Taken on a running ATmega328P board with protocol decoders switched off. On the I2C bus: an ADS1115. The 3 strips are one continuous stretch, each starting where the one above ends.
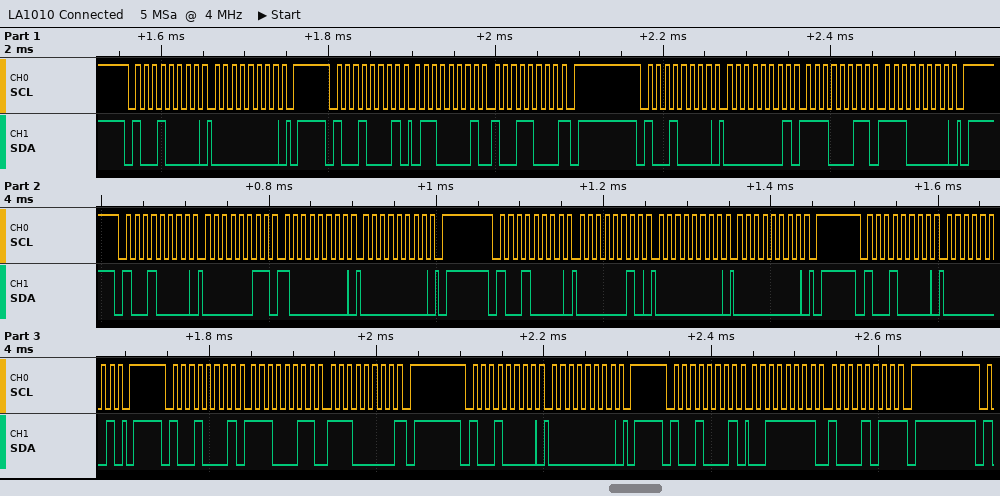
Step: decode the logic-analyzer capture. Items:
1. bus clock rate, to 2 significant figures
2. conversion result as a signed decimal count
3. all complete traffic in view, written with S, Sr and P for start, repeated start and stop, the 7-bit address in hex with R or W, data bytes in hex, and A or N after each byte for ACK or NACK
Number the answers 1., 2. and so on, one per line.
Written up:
1. 100 kHz
2. 24984
3. S 48W A 00 A P S 48R A 61 A 98 N P S 48W A 01 A E3 A E0 A P S 48W A 03 A 80 A 00 A P S 48W A 02 A 00 A 00 A P S 48W A 01 A P S 48R A E3 A E0 N P S 48W A 00 A P S 48R A 3F A 8B N P
